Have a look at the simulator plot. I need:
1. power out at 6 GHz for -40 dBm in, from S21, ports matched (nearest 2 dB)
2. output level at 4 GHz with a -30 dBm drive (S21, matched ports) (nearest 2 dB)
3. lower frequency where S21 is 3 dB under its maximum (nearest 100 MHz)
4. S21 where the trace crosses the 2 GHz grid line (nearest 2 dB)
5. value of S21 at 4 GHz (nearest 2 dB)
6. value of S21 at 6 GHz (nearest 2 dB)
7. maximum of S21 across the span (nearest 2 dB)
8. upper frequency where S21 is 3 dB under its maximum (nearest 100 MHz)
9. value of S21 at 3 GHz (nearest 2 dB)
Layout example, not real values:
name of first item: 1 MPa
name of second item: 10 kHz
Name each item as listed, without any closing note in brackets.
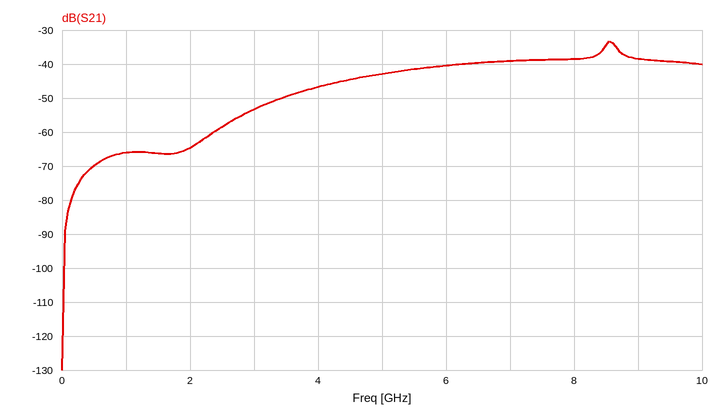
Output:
power out at 6 GHz for -40 dBm in, from S21, ports matched: -80 dBm
output level at 4 GHz with a -30 dBm drive (S21, matched ports): -76 dBm
lower frequency where S21 is 3 dB under its maximum: 8.4 GHz
S21 where the trace crosses the 2 GHz grid line: -64 dB
value of S21 at 4 GHz: -46 dB
value of S21 at 6 GHz: -40 dB
maximum of S21 across the span: -34 dB
upper frequency where S21 is 3 dB under its maximum: 8.7 GHz
value of S21 at 3 GHz: -54 dB
